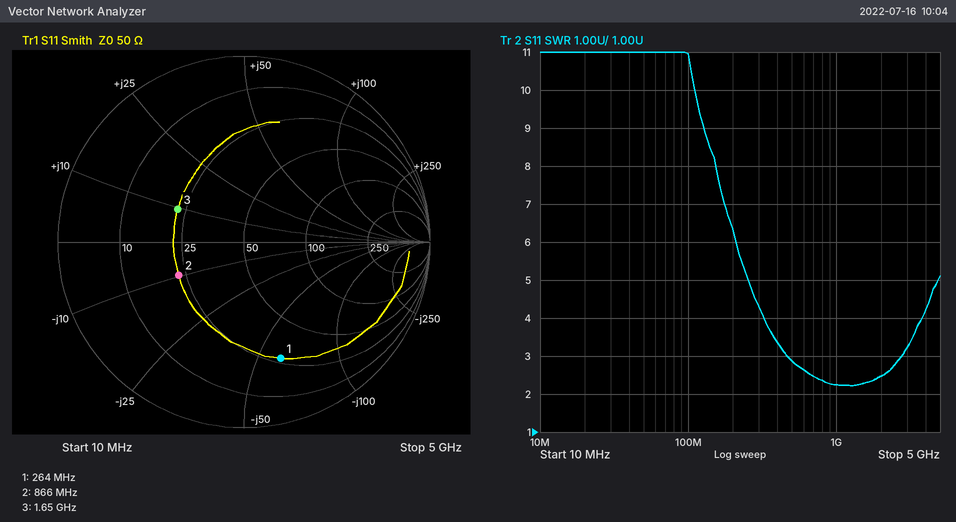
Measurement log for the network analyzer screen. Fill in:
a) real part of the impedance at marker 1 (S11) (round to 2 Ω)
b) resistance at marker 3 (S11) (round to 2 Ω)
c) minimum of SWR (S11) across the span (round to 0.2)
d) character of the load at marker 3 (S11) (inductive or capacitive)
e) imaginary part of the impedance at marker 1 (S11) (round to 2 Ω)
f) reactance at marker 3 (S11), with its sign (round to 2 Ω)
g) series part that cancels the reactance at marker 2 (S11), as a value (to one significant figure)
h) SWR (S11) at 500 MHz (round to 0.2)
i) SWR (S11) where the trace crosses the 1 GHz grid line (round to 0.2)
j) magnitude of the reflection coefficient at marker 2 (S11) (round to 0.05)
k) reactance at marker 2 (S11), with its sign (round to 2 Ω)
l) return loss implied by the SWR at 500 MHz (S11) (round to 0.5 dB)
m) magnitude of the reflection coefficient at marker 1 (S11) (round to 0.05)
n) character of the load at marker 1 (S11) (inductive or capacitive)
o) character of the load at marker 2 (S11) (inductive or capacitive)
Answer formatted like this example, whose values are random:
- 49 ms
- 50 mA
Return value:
- 28 Ω
- 22 Ω
- 2.2
- inductive
- -60 Ω
- +10 Ω
- 2 nH
- 2.8
- 2.2
- 0.40
- -10 Ω
- 6.5 dB
- 0.65
- capacitive
- capacitive
